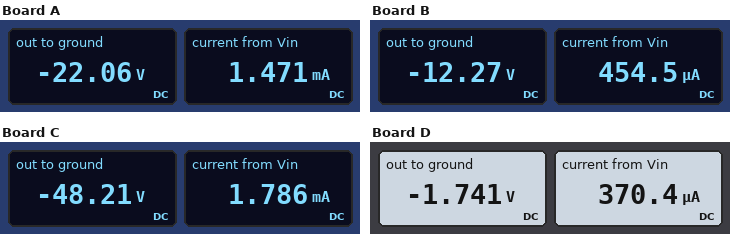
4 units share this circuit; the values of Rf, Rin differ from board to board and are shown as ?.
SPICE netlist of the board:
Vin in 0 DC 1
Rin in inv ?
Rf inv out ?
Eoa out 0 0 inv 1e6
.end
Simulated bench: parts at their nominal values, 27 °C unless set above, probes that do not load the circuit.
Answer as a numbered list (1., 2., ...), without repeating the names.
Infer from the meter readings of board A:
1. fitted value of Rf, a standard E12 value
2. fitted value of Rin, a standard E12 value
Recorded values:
1. 15 kΩ
2. 680 Ω
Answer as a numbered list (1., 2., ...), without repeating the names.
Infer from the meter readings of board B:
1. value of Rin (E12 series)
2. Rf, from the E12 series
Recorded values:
1. 2.2 kΩ
2. 27 kΩ
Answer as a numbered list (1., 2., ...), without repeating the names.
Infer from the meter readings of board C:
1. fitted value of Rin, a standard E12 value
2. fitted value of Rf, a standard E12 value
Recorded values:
1. 560 Ω
2. 27 kΩ
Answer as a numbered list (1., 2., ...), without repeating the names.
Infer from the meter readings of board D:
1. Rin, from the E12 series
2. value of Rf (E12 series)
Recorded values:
1. 2.7 kΩ
2. 4.7 kΩ
